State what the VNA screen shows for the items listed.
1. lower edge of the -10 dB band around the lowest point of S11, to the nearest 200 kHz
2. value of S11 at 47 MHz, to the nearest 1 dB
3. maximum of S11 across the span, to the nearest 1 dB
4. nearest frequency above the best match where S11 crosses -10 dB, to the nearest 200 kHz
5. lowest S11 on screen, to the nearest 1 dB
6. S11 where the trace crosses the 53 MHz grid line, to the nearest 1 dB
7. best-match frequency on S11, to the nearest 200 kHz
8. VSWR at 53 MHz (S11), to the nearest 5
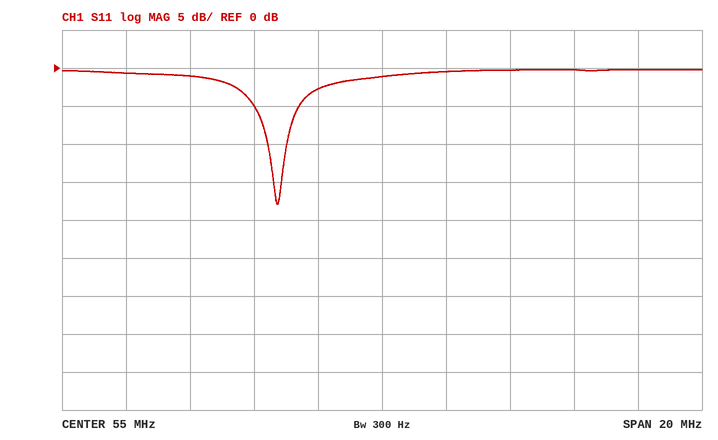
51.4 MHz
-1 dB
0 dB
52.0 MHz
-18 dB
-3 dB
51.8 MHz
5
